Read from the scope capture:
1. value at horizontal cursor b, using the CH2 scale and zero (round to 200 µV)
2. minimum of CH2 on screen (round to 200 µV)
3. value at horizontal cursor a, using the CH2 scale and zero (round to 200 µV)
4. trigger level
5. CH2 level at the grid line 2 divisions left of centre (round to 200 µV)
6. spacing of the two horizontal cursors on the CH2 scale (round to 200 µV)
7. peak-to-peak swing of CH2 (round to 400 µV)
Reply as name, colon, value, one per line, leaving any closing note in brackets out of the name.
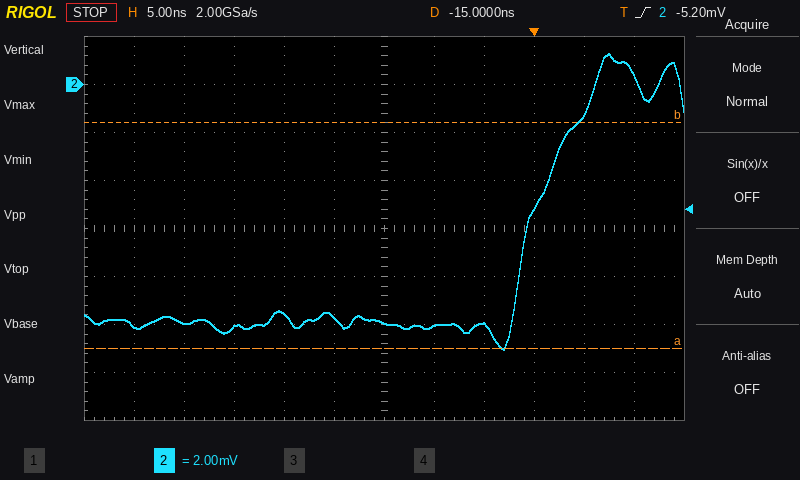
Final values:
value at horizontal cursor b, using the CH2 scale and zero: -1.6 mV
minimum of CH2 on screen: -11.0 mV
value at horizontal cursor a, using the CH2 scale and zero: -11.0 mV
trigger level: -5.20 mV
CH2 level at the grid line 2 divisions left of centre: -9.6 mV
spacing of the two horizontal cursors on the CH2 scale: 9.4 mV
peak-to-peak swing of CH2: 12.4 mV
